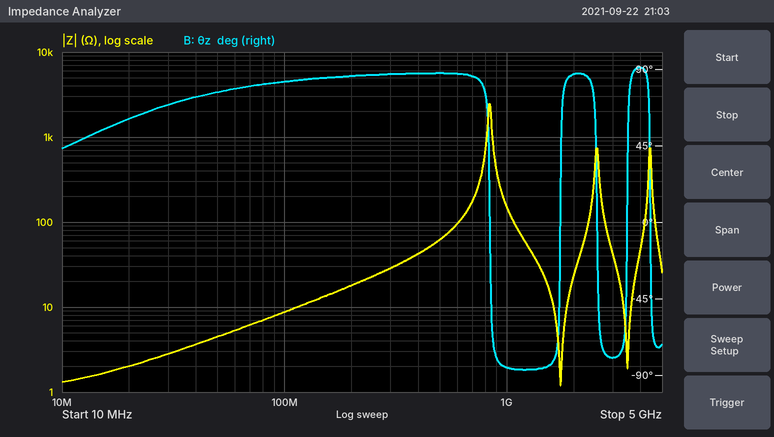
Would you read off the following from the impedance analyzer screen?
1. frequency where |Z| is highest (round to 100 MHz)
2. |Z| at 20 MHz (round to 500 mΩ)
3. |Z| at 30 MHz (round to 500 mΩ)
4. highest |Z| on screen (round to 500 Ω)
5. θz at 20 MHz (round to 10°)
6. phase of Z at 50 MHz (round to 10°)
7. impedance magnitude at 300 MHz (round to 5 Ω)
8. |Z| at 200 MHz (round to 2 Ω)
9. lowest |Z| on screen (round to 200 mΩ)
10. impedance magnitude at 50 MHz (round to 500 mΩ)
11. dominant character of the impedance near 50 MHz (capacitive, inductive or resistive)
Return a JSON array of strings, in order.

["800 MHz", "2.0 Ω", "3.0 Ω", "2.5 kΩ", "60°", "80°", "30 Ω", "18 Ω", "1.2 Ω", "4.5 Ω", "inductive"]
